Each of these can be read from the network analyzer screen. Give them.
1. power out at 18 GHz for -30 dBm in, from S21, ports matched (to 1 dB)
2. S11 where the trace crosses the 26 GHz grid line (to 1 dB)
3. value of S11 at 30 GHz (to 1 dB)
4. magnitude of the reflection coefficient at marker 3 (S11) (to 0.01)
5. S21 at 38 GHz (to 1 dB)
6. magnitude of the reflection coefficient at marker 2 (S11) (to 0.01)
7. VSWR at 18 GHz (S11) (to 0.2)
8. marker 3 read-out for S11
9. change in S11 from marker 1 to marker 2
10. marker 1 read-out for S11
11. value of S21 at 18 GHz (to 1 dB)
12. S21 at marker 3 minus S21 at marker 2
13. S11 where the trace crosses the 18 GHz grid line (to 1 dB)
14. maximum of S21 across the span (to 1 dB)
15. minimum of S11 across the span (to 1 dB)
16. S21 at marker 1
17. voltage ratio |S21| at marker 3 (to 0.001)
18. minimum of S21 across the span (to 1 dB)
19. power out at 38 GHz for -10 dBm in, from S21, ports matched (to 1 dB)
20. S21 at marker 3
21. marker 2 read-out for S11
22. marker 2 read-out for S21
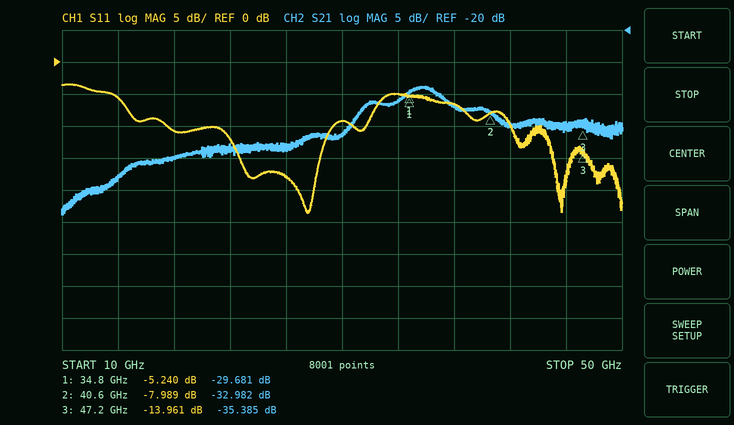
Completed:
-70 dBm
-18 dB
-9 dB
0.20
-32 dB
0.40
1.8
-13.961 dB
-2.749 dB
-5.240 dB
-40 dB
-2.403 dB
-11 dB
-29 dB
-24 dB
-29.681 dB
0.017
-49 dB
-42 dBm
-35.385 dB
-7.989 dB
-32.982 dB
